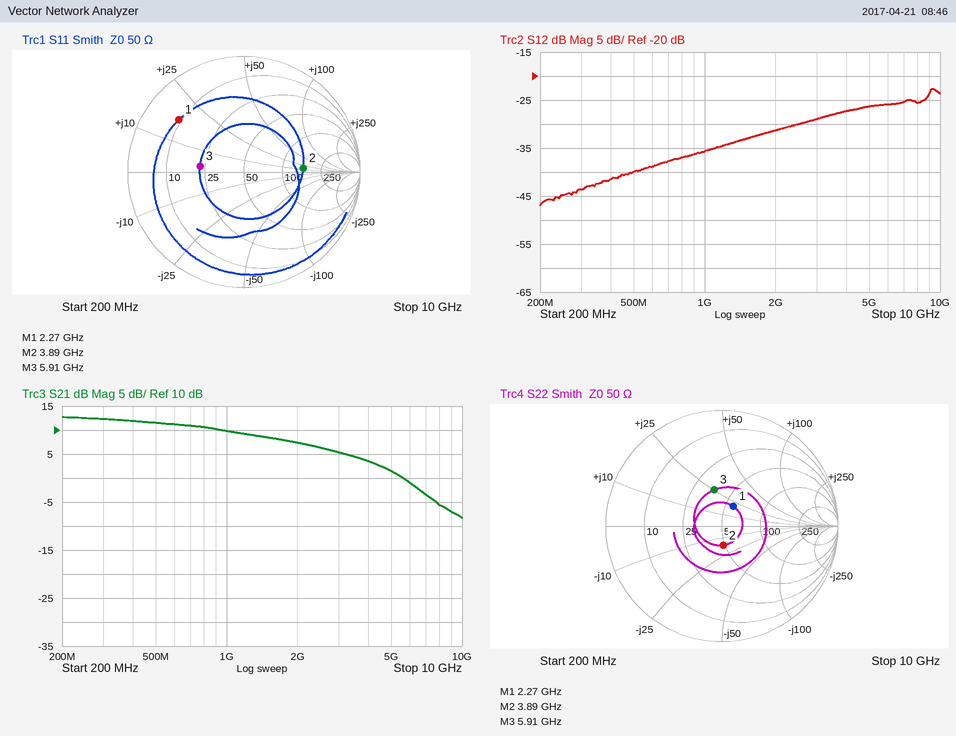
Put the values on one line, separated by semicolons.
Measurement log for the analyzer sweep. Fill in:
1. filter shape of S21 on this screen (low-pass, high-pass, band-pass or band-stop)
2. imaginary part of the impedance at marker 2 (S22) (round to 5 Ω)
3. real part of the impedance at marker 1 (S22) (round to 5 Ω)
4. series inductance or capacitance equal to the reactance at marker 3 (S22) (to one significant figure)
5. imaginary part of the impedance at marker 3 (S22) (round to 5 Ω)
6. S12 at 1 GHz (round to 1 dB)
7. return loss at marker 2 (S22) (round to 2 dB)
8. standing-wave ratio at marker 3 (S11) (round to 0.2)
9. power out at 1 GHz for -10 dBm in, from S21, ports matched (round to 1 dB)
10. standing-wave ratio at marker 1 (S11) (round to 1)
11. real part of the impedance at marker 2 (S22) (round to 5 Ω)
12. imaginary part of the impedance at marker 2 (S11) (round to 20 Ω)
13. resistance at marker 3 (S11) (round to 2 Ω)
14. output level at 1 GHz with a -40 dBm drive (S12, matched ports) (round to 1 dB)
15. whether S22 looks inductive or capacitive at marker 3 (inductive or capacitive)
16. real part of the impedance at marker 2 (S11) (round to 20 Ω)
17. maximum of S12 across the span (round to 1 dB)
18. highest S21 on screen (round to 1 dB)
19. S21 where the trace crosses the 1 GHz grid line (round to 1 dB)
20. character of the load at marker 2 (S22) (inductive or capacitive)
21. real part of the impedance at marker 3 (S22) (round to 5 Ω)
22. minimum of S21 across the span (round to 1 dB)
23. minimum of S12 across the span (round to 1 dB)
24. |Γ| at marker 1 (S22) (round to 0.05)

low-pass; -15 Ω; 55 Ω; 700 pH; +25 Ω; -36 dB; 16 dB; 2.2; 0 dBm; 6; 50 Ω; +20 Ω; 22 Ω; -76 dBm; inductive; 160 Ω; -23 dB; 13 dB; 10 dB; capacitive; 35 Ω; -8 dB; -47 dB; 0.20
